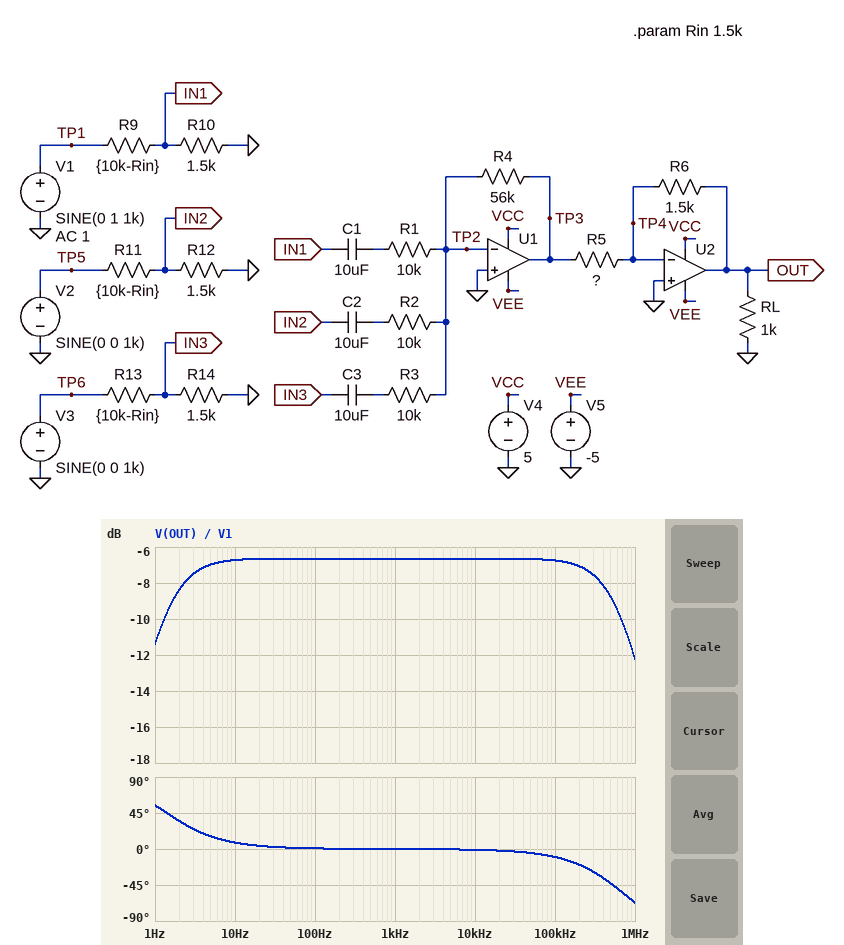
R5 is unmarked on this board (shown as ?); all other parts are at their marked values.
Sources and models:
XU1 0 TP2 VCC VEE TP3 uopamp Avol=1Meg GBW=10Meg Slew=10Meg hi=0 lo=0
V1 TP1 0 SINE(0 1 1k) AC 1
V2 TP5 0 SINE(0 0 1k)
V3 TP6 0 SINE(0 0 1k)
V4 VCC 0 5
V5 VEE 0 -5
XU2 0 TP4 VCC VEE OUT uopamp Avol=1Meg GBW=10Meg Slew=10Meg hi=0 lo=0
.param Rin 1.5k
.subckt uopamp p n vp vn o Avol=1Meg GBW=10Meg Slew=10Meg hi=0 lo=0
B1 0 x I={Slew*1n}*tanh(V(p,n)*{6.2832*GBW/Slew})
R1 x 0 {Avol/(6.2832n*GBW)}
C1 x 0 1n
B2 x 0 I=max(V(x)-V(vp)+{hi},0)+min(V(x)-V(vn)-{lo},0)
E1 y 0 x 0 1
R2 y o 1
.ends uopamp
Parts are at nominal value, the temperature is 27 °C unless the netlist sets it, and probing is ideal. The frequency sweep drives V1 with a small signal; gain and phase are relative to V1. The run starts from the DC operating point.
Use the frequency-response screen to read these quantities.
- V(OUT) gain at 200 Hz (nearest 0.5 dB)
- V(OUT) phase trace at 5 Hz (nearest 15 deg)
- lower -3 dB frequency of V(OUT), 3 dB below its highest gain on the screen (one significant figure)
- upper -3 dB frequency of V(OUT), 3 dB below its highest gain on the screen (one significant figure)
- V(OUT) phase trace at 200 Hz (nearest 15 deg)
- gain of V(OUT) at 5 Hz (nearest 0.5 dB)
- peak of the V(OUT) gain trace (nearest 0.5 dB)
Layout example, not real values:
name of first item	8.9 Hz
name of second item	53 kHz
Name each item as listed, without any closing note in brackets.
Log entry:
V(OUT) gain at 200 Hz	-6.5 dB
V(OUT) phase trace at 5 Hz	15 deg
lower -3 dB frequency of V(OUT), 3 dB below its highest gain on the screen	1 Hz
upper -3 dB frequency of V(OUT), 3 dB below its highest gain on the screen	600 kHz
V(OUT) phase trace at 200 Hz	0 deg
gain of V(OUT) at 5 Hz	-7.0 dB
peak of the V(OUT) gain trace	-6.5 dB
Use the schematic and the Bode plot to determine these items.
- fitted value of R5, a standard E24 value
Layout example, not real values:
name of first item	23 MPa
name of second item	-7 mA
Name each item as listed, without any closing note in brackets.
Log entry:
fitted value of R5, a standard E24 value	2.4 kΩ
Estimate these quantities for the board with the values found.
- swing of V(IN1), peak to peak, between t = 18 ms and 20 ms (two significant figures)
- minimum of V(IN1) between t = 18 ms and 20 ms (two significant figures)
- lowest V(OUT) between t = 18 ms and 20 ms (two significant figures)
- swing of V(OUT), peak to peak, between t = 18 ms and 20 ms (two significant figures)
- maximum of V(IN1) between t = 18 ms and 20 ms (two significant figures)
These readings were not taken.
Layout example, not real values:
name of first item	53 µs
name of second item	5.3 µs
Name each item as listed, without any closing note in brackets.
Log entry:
swing of V(IN1), peak to peak, between t = 18 ms and 20 ms	270 mV
minimum of V(IN1) between t = 18 ms and 20 ms	-130 mV
lowest V(OUT) between t = 18 ms and 20 ms	-470 mV
swing of V(OUT), peak to peak, between t = 18 ms and 20 ms	930 mV
maximum of V(IN1) between t = 18 ms and 20 ms	130 mV
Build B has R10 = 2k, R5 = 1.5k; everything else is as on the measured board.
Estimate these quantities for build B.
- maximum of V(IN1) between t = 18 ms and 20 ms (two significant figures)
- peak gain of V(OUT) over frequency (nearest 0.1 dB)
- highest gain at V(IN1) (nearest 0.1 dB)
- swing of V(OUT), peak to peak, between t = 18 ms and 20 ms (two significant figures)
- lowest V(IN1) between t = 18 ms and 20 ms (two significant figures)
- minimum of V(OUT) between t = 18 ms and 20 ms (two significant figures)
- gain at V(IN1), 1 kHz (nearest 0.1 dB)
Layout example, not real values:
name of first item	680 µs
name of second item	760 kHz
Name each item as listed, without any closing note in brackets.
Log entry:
maximum of V(IN1) between t = 18 ms and 20 ms	160 mV
peak gain of V(OUT) over frequency	-0.7 dB
highest gain at V(IN1)	-14.4 dB
swing of V(OUT), peak to peak, between t = 18 ms and 20 ms	1.8 V
lowest V(IN1) between t = 18 ms and 20 ms	-160 mV
minimum of V(OUT) between t = 18 ms and 20 ms	-920 mV
gain at V(IN1), 1 kHz	-15.7 dB
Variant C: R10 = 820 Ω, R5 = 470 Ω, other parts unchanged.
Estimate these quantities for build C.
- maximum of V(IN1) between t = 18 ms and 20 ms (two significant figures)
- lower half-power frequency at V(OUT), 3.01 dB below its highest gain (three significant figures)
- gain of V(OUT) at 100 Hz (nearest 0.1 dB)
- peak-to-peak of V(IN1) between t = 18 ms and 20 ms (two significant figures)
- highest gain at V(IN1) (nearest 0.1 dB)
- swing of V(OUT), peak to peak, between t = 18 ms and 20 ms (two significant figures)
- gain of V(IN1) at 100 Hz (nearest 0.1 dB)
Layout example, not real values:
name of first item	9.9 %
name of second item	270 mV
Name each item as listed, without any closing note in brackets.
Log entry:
maximum of V(IN1) between t = 18 ms and 20 ms	82 mV
lower half-power frequency at V(OUT), 3.01 dB below its highest gain	1.48 Hz
gain of V(OUT) at 100 Hz	3.3 dB
peak-to-peak of V(IN1) between t = 18 ms and 20 ms	160 mV
highest gain at V(IN1)	-21.1 dB
swing of V(OUT), peak to peak, between t = 18 ms and 20 ms	2.9 V
gain of V(IN1) at 100 Hz	-21.7 dB
